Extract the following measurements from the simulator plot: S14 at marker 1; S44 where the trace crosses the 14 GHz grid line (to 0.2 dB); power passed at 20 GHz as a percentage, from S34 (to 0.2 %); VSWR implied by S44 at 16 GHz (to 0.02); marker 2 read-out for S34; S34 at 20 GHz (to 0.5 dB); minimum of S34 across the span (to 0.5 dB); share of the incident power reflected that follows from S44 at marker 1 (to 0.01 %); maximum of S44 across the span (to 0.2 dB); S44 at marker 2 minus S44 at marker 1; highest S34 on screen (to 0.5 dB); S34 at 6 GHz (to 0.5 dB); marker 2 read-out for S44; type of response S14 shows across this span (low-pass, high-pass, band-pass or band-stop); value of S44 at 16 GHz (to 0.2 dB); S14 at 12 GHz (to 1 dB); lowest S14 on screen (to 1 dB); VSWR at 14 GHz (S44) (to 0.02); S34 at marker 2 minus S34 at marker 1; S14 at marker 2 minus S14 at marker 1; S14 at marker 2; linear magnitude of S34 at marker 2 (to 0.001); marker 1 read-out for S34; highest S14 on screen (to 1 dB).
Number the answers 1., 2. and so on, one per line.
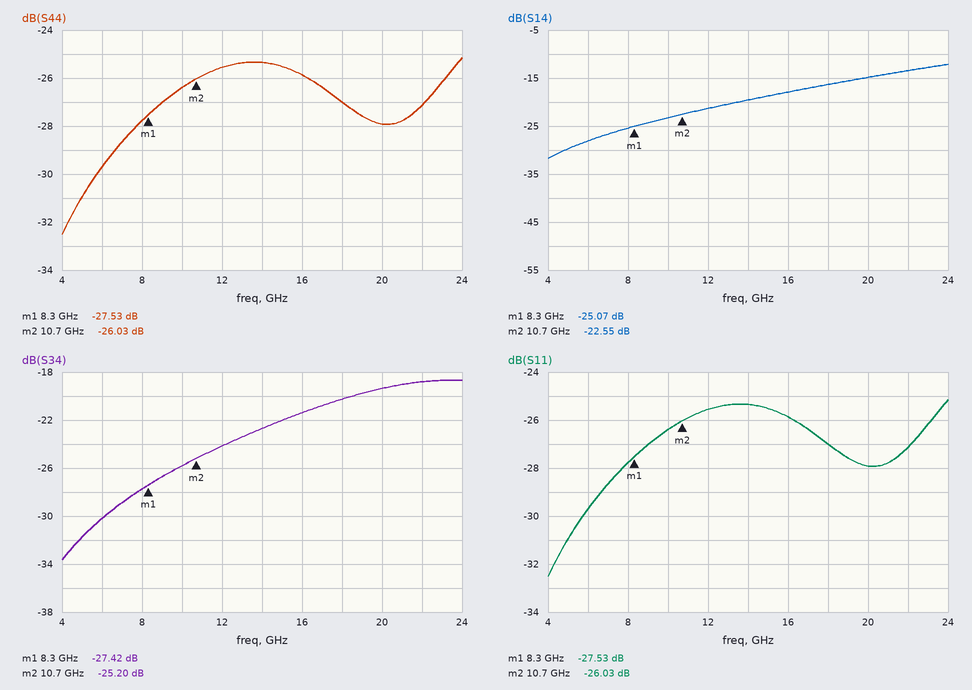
1. -25.07 dB
2. -25.4 dB
3. 1.2 %
4. 1.10
5. -25.20 dB
6. -19.5 dB
7. -33.5 dB
8. 0.18 %
9. -25.2 dB
10. 1.50 dB
11. -18.5 dB
12. -30.0 dB
13. -26.03 dB
14. high-pass
15. -25.8 dB
16. -21 dB
17. -32 dB
18. 1.12
19. 2.22 dB
20. 2.52 dB
21. -22.55 dB
22. 0.055
23. -27.42 dB
24. -12 dB
